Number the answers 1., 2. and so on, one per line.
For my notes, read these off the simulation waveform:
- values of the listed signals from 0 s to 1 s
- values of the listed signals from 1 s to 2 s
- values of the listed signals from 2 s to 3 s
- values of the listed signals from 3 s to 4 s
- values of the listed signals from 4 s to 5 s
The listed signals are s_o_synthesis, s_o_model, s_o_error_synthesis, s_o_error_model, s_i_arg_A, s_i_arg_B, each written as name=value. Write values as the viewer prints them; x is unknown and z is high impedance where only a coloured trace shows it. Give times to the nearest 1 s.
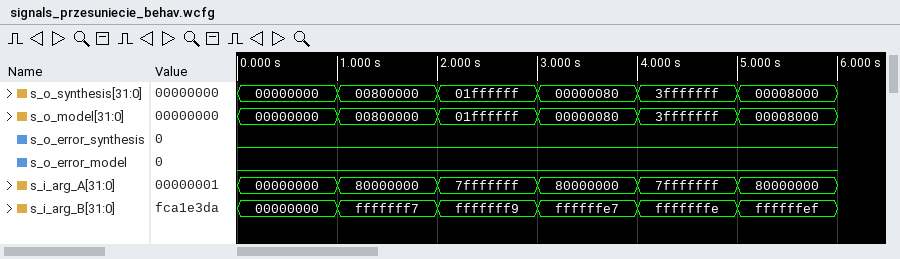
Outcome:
1. s_o_synthesis=00000000, s_o_model=00000000, s_o_error_synthesis=0, s_o_error_model=0, s_i_arg_A=00000000, s_i_arg_B=00000000
2. s_o_synthesis=00800000, s_o_model=00800000, s_o_error_synthesis=0, s_o_error_model=0, s_i_arg_A=80000000, s_i_arg_B=fffffff7
3. s_o_synthesis=01ffffff, s_o_model=01ffffff, s_o_error_synthesis=0, s_o_error_model=0, s_i_arg_A=7fffffff, s_i_arg_B=fffffff9
4. s_o_synthesis=00000080, s_o_model=00000080, s_o_error_synthesis=0, s_o_error_model=0, s_i_arg_A=80000000, s_i_arg_B=ffffffe7
5. s_o_synthesis=3fffffff, s_o_model=3fffffff, s_o_error_synthesis=0, s_o_error_model=0, s_i_arg_A=7fffffff, s_i_arg_B=fffffffe
